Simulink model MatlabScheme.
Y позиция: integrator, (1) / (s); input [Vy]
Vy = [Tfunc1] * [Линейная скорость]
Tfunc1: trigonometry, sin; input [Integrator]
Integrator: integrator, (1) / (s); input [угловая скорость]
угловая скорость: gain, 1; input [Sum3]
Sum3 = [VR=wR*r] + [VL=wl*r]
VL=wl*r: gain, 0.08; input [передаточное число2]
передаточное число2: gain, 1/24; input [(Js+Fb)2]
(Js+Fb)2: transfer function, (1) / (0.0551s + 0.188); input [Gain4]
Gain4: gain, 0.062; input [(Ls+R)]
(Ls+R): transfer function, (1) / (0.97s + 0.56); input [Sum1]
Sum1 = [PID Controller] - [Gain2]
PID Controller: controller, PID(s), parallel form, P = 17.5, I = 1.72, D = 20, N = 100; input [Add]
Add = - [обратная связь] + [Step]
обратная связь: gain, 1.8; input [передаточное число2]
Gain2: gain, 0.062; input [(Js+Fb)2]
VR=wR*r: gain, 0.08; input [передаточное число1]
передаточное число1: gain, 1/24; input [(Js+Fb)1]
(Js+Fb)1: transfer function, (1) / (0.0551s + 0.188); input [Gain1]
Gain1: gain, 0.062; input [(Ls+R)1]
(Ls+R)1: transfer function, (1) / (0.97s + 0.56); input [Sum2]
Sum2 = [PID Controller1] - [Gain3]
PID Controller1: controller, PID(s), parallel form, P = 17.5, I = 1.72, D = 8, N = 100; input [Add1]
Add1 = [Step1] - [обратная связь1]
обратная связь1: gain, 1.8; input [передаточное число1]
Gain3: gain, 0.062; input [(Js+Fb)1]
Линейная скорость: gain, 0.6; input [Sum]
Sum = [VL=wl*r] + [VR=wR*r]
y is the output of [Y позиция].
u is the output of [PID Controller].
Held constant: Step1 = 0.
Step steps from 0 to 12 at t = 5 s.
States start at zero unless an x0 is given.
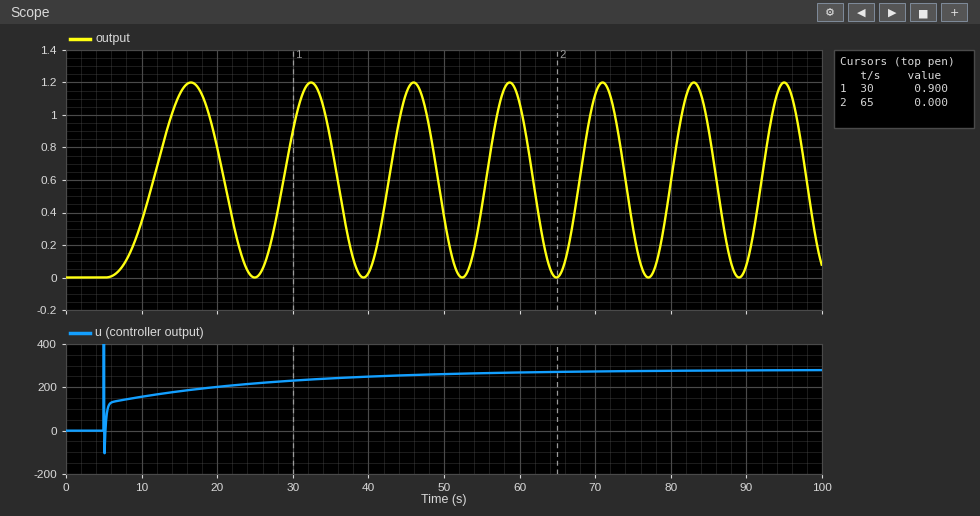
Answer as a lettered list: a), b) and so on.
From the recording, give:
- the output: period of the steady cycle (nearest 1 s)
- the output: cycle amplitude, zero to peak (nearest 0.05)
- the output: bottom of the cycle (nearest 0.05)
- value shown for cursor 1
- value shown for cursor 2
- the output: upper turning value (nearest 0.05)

a) 12 s
b) 0.60
c) 0.00
d) 0.900
e) 0.000
f) 1.20
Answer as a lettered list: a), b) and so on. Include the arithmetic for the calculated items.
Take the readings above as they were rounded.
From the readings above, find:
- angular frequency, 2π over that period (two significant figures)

a) 2π / 12 = 0.52 rad/s
